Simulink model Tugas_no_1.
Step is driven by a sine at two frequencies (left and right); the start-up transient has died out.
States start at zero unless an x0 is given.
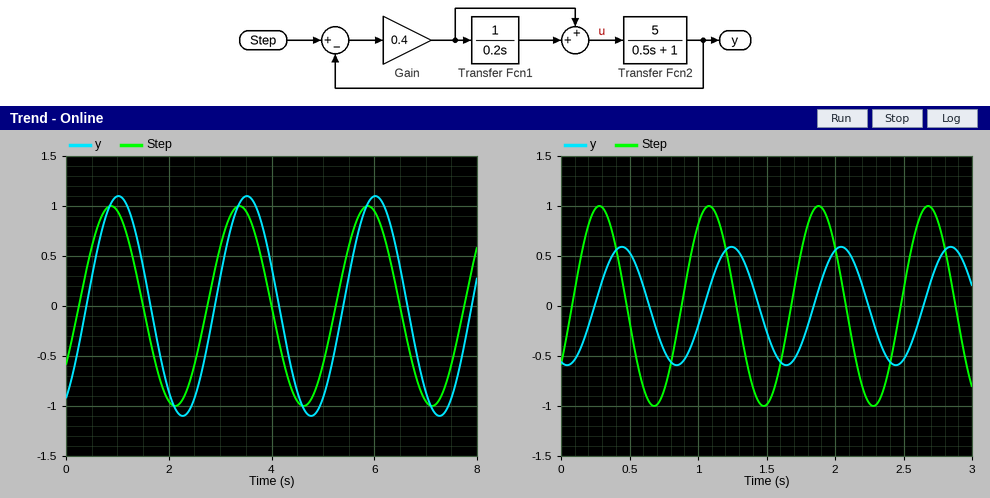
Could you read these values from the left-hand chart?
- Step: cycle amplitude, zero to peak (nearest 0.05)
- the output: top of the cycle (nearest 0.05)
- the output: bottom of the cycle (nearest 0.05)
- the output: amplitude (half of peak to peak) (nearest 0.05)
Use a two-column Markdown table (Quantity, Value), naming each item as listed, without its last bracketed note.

| Quantity | Value |
|---|---|
| Step: cycle amplitude, zero to peak | 1.00 |
| the output: top of the cycle | 1.10 |
| the output: bottom of the cycle | -1.10 |
| the output: amplitude (half of peak to peak) | 1.10 |
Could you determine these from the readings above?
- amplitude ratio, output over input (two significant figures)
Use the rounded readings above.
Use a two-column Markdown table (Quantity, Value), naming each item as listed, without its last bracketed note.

| Quantity | Value |
|---|---|
| amplitude ratio, output over input | 1.1 |
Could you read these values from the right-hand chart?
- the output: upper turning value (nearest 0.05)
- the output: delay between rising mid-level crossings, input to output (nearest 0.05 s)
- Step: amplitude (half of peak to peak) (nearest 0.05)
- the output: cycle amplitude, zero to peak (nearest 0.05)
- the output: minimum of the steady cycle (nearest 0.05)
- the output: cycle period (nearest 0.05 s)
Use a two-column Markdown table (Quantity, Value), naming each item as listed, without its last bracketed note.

| Quantity | Value |
|---|---|
| the output: upper turning value | 0.60 |
| the output: delay between rising mid-level crossings, input to output | 0.15 s |
| Step: amplitude (half of peak to peak) | 1.00 |
| the output: cycle amplitude, zero to peak | 0.60 |
| the output: minimum of the steady cycle | -0.60 |
| the output: cycle period | 0.80 s |
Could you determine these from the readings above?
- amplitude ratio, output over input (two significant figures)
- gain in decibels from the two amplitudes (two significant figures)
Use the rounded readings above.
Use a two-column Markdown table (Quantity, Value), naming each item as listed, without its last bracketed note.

| Quantity | Value |
|---|---|
| amplitude ratio, output over input | 0.60 |
| gain in decibels from the two amplitudes | -4.4 dB |
